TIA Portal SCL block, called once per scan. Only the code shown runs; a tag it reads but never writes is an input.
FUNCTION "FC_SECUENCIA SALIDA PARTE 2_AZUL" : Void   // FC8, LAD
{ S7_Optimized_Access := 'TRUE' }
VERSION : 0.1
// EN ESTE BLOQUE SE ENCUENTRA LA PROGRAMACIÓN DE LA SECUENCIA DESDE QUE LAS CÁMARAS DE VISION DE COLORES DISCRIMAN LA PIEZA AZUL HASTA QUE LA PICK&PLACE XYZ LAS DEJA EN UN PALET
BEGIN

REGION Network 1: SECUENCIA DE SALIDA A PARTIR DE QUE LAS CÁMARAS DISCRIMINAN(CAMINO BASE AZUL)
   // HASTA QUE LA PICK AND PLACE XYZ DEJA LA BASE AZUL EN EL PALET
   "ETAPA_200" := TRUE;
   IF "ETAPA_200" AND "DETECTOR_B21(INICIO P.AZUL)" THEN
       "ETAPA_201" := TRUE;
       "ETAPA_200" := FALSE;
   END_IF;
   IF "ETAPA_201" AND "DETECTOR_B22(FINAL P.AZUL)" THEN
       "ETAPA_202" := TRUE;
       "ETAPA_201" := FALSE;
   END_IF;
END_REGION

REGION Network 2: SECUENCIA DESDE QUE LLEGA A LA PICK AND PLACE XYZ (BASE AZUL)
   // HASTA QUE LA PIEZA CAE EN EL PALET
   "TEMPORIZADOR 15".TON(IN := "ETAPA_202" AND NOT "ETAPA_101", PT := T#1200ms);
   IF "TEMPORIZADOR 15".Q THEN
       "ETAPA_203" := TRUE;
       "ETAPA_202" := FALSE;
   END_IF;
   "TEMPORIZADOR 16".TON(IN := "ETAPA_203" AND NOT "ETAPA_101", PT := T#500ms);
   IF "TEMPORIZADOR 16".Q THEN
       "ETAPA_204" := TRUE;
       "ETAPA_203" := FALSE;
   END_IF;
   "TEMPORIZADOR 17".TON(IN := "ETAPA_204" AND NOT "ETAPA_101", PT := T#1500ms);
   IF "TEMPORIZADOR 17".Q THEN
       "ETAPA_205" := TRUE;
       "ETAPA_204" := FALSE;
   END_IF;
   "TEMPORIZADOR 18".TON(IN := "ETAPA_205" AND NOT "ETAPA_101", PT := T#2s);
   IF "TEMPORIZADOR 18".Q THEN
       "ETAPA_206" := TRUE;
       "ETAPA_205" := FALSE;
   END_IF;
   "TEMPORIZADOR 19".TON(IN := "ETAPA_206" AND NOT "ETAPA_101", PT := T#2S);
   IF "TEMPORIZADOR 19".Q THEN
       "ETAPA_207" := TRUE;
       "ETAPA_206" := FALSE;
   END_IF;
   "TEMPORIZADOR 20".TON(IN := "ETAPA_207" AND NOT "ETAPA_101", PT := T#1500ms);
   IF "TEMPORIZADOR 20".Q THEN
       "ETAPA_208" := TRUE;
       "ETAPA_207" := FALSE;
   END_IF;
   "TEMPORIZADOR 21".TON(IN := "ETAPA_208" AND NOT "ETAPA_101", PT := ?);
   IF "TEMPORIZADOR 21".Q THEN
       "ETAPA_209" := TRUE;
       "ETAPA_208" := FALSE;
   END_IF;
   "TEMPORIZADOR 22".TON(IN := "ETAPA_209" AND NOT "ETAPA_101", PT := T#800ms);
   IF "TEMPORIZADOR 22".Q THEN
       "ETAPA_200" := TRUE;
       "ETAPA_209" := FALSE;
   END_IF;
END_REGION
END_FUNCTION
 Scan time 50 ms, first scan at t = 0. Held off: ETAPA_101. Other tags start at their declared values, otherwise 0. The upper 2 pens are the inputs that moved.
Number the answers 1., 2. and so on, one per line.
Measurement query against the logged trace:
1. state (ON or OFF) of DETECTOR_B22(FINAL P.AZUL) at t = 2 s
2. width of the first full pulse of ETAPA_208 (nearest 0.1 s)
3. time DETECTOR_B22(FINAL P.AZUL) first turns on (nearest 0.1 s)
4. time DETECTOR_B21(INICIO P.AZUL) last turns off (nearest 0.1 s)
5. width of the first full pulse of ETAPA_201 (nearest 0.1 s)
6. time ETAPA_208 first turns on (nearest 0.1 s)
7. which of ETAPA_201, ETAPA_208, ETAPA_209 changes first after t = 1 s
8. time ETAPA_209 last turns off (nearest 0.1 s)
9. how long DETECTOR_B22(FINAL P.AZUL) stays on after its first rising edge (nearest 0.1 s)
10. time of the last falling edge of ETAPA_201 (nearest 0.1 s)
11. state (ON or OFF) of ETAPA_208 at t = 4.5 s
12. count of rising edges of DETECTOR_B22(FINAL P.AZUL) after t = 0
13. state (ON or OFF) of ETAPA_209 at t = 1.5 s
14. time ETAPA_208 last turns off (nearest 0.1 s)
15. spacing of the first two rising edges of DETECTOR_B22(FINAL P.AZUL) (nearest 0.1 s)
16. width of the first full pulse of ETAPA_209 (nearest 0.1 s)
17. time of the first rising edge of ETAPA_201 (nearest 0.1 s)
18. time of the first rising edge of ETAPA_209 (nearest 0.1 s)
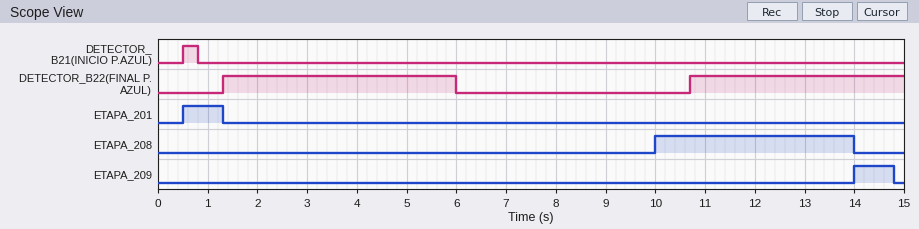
1. ON
2. 4.0 s
3. 1.3 s
4. 0.8 s
5. 0.8 s
6. 10.0 s
7. ETAPA_201
8. 14.8 s
9. 4.7 s
10. 1.3 s
11. OFF
12. 2
13. OFF
14. 14.0 s
15. 9.4 s
16. 0.8 s
17. 0.5 s
18. 14.0 s
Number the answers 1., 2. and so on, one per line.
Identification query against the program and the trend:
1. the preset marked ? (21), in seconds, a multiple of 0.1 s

1. 4.0 s
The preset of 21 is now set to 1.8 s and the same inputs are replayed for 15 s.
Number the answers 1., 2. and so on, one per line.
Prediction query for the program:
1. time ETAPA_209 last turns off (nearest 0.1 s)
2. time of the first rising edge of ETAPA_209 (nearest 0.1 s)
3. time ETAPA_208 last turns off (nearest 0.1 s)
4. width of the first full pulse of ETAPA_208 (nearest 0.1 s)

1. 12.6 s
2. 11.8 s
3. 11.8 s
4. 1.8 s
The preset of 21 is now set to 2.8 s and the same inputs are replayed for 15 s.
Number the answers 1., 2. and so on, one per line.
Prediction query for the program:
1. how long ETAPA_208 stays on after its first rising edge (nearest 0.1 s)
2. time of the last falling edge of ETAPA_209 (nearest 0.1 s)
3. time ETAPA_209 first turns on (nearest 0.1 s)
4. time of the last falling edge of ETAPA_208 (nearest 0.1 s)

1. 2.8 s
2. 13.6 s
3. 12.8 s
4. 12.8 s
